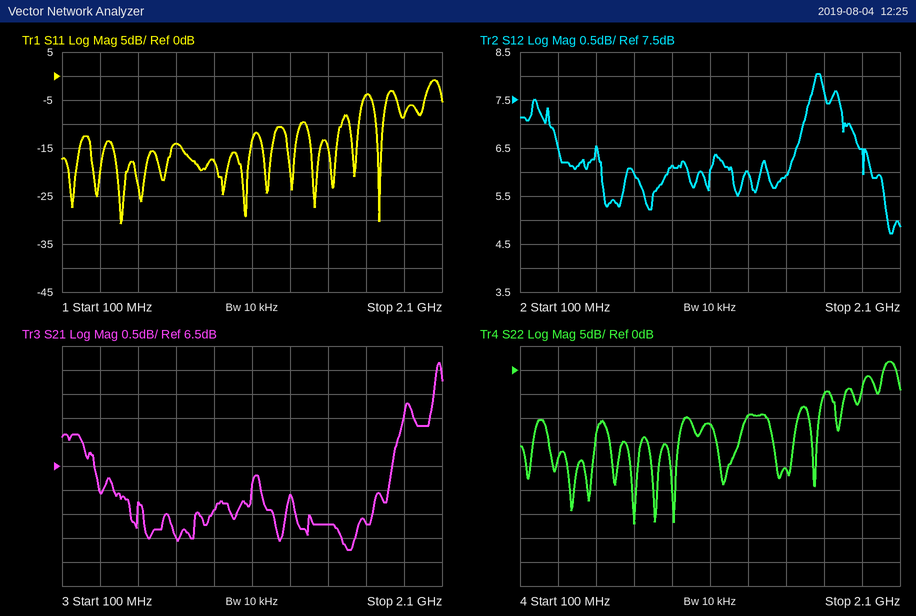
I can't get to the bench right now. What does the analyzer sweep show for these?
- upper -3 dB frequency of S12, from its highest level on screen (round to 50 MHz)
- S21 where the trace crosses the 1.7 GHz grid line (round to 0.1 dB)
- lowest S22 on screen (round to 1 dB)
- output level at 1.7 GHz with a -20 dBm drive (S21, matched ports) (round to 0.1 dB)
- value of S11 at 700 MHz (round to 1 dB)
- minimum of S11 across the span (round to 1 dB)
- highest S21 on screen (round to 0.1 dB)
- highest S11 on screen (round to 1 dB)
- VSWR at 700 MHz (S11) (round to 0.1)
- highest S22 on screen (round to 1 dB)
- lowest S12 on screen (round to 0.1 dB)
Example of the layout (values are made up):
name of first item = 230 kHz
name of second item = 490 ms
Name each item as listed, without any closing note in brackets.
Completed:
upper -3 dB frequency of S12, from its highest level on screen = 2.05 GHz
S21 where the trace crosses the 1.7 GHz grid line = 5.3 dB
lowest S22 on screen = -32 dB
output level at 1.7 GHz with a -20 dBm drive (S21, matched ports) = -14.7 dBm
value of S11 at 700 MHz = -14 dB
minimum of S11 across the span = -31 dB
highest S21 on screen = 8.7 dB
highest S11 on screen = -1 dB
VSWR at 700 MHz (S11) = 1.5
highest S22 on screen = 2 dB
lowest S12 on screen = 4.7 dB
